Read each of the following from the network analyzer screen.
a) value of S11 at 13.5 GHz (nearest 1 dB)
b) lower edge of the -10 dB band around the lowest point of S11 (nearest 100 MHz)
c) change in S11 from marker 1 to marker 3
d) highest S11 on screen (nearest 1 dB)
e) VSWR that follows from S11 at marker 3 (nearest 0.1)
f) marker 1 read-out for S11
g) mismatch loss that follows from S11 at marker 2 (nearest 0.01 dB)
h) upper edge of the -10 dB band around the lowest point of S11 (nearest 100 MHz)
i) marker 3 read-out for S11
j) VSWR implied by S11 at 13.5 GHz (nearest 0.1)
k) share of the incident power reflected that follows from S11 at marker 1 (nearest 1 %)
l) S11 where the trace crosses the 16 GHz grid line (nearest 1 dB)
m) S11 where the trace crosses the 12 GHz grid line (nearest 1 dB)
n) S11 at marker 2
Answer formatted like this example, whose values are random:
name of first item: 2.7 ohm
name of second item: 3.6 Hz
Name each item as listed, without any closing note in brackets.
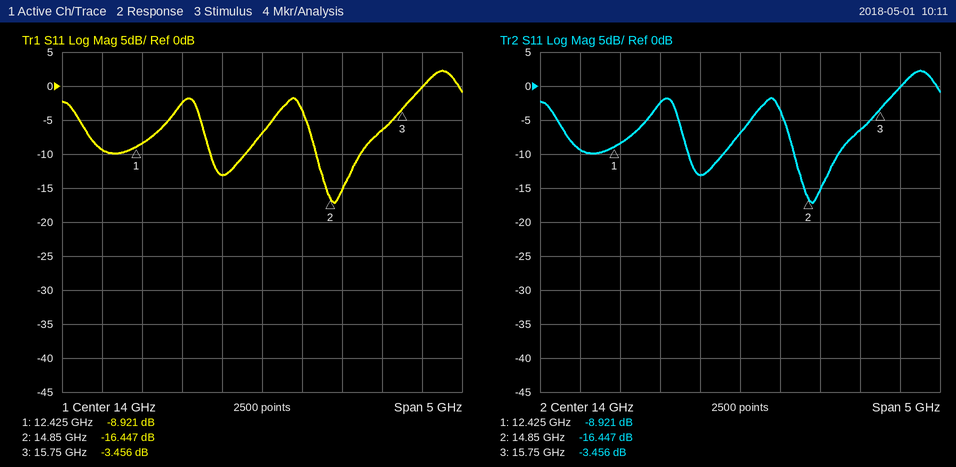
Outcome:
value of S11 at 13.5 GHz: -13 dB
lower edge of the -10 dB band around the lowest point of S11: 14.7 GHz
change in S11 from marker 1 to marker 3: 5.465 dB
highest S11 on screen: 2 dB
VSWR that follows from S11 at marker 3: 5.1
marker 1 read-out for S11: -8.921 dB
mismatch loss that follows from S11 at marker 2: 0.10 dB
upper edge of the -10 dB band around the lowest point of S11: 15.2 GHz
marker 3 read-out for S11: -3.456 dB
VSWR implied by S11 at 13.5 GHz: 1.6
share of the incident power reflected that follows from S11 at marker 1: 13 %
S11 where the trace crosses the 16 GHz grid line: 0 dB
S11 where the trace crosses the 12 GHz grid line: -9 dB
S11 at marker 2: -16.447 dB
